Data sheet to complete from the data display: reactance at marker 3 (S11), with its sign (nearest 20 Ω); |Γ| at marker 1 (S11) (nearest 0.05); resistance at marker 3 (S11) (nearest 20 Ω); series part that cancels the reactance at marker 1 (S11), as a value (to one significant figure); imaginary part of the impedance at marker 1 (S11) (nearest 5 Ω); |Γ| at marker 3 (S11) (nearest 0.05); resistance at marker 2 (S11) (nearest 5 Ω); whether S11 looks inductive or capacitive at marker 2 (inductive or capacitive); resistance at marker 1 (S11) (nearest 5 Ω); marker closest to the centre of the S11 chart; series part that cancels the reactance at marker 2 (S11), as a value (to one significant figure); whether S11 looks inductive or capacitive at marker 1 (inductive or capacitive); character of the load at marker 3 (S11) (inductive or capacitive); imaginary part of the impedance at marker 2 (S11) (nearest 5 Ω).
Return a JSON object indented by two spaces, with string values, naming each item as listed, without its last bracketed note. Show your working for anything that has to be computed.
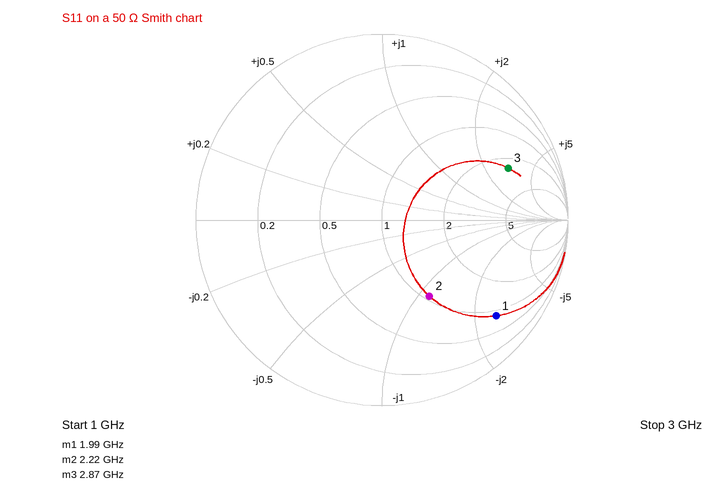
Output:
{
  "reactance at marker 3 (S11), with its sign": "+160 Ω",
  "|Γ| at marker 1 (S11)": "0.80",
  "resistance at marker 3 (S11)": "120 Ω",
  "series part that cancels the reactance at marker 1 (S11), as a value": "L = 125 Ω/(2π × 1.99 GHz) ≈ 10 nH",
  "imaginary part of the impedance at marker 1 (S11)": "-125 Ω",
  "|Γ| at marker 3 (S11)": "0.75",
  "resistance at marker 2 (S11)": "55 Ω",
  "whether S11 looks inductive or capacitive at marker 2": "capacitive",
  "resistance at marker 1 (S11)": "45 Ω",
  "marker closest to the centre of the S11 chart": "marker 2",
  "series part that cancels the reactance at marker 2 (S11), as a value": "L = 55 Ω/(2π × 2.22 GHz) ≈ 4 nH",
  "whether S11 looks inductive or capacitive at marker 1": "capacitive",
  "character of the load at marker 3 (S11)": "inductive",
  "imaginary part of the impedance at marker 2 (S11)": "-55 Ω"
}
